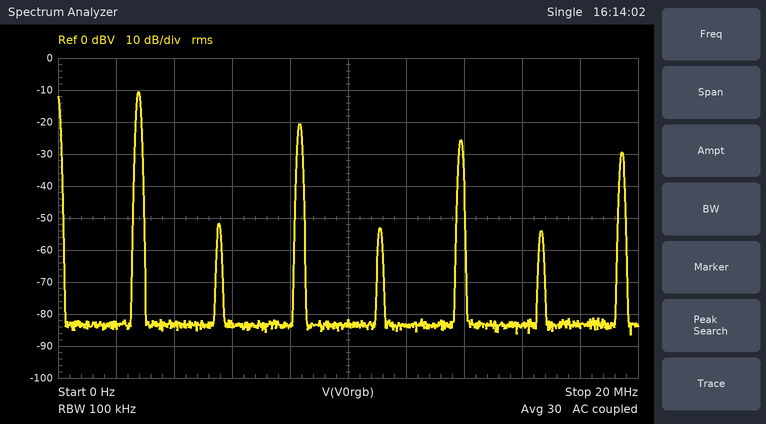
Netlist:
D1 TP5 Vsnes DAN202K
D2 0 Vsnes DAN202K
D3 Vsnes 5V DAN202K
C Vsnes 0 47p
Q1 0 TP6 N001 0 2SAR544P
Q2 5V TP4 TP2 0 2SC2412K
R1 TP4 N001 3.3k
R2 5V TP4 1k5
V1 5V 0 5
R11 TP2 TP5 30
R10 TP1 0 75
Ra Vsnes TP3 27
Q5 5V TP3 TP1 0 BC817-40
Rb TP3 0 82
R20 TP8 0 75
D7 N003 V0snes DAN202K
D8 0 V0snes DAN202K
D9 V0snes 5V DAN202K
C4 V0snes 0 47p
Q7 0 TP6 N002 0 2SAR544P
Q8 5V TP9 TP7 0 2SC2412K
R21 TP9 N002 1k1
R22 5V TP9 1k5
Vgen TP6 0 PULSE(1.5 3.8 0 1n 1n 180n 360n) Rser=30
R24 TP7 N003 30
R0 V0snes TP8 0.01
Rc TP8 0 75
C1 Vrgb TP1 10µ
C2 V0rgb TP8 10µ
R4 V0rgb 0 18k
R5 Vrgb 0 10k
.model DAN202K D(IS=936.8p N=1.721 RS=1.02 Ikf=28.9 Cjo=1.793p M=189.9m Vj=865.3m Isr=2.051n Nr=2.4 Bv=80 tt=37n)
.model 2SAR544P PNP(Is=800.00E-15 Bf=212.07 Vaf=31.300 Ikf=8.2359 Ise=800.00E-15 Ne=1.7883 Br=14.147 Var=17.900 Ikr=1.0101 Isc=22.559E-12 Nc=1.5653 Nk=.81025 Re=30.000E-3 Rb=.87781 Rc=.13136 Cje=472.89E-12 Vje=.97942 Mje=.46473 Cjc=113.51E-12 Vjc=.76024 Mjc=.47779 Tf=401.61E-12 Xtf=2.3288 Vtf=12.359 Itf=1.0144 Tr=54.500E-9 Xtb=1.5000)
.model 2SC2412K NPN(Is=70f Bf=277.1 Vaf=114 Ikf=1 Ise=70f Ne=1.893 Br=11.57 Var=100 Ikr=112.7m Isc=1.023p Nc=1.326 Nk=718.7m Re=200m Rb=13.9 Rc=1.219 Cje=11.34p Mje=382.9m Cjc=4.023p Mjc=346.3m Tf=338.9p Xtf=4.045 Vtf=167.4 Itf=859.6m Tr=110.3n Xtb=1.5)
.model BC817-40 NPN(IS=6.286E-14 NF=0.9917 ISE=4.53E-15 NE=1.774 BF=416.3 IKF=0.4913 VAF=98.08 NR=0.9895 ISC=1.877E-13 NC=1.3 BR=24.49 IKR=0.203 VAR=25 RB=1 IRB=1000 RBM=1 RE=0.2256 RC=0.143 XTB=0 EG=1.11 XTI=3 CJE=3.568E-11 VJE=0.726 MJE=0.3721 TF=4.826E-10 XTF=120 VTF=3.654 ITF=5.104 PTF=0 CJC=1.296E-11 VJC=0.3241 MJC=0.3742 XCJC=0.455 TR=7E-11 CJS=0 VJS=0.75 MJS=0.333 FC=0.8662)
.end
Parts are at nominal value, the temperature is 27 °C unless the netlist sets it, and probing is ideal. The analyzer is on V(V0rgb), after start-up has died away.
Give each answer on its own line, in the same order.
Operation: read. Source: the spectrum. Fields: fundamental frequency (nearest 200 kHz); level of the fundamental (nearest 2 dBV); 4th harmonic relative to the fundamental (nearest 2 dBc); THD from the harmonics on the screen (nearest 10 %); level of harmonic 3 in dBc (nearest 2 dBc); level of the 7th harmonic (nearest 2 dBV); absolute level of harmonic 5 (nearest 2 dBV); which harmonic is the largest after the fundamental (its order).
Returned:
2.8 MHz
-10 dBV
-42 dBc
40 %
-10 dBc
-30 dBV
-26 dBV
3
